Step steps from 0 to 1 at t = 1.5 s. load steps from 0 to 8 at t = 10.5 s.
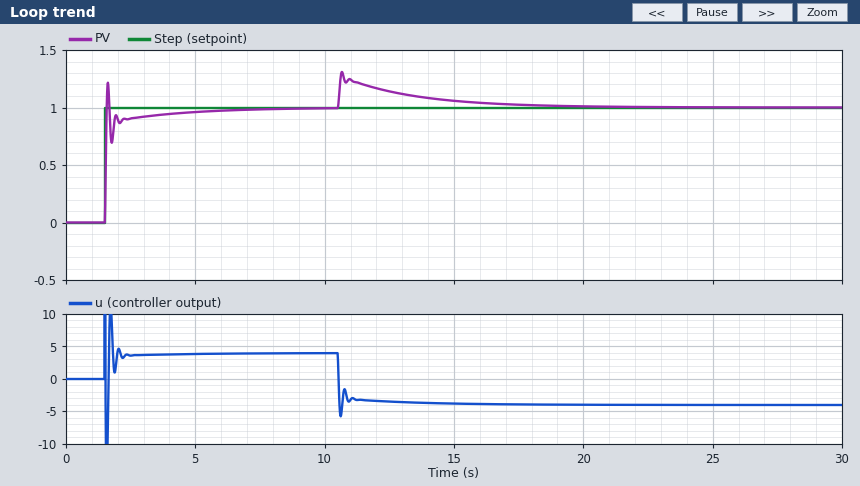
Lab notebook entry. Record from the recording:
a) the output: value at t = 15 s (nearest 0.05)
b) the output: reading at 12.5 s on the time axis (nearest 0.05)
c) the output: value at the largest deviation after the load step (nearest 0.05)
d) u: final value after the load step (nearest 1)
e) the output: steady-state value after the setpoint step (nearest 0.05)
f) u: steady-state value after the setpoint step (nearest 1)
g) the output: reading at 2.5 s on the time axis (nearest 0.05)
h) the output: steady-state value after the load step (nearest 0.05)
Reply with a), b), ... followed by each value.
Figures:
a) 1.05
b) 1.15
c) 1.30
d) -4
e) 1.00
f) 4
g) 0.90
h) 1.00
